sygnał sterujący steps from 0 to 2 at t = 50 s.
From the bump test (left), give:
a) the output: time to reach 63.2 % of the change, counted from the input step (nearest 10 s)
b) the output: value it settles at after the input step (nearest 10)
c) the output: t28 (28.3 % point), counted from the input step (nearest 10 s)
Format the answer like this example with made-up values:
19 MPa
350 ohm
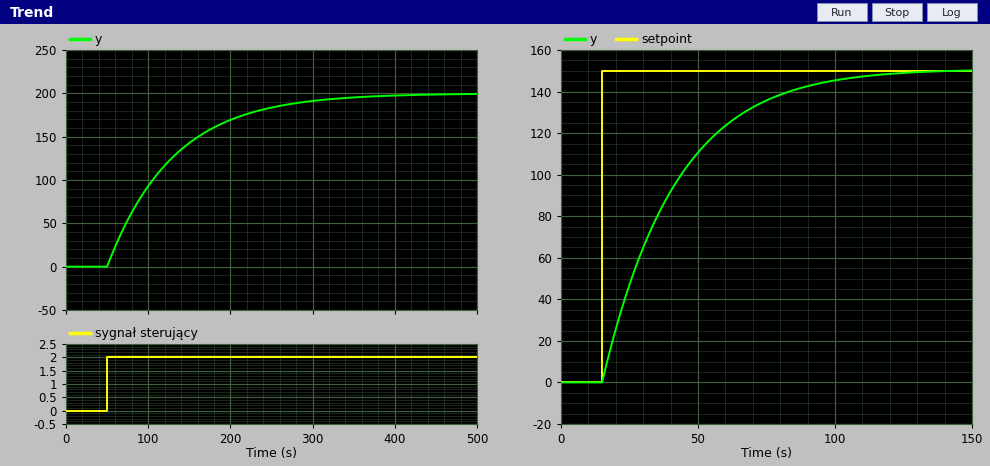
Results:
80 s
200
30 s
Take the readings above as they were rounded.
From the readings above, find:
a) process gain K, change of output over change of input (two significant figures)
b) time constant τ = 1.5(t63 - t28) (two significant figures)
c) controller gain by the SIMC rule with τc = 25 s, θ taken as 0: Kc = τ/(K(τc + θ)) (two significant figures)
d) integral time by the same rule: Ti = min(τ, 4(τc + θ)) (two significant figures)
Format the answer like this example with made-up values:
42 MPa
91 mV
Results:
100
75 s
0.030
75 s
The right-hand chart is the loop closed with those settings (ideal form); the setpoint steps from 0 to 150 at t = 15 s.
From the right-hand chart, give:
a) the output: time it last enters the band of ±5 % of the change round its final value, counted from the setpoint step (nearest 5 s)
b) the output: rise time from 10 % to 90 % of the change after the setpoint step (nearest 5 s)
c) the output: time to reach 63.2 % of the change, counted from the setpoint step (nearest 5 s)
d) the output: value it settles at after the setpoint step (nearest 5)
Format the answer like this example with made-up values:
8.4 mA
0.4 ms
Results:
75 s
55 s
25 s
150
